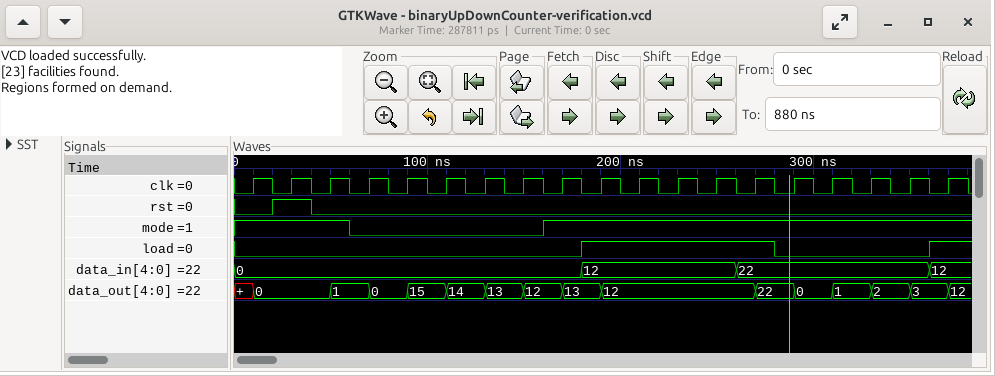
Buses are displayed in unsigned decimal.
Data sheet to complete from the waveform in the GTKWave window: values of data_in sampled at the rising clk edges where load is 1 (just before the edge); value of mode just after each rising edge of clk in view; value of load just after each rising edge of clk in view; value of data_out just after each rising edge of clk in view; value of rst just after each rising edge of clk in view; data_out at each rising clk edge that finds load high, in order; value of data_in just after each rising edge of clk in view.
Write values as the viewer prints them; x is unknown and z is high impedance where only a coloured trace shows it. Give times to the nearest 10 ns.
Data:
12, 12, 12, 12, 22, 12
1 1 1 0 0 0 0 0 1 1 1 1 1 1 1 1 1 1 1
0 0 0 0 0 0 0 0 0 1 1 1 1 1 0 0 0 0 1
0, 0, 1, 0, 15, 14, 13, 12, 13, 12, 12, 12, 12, 22, 0, 1, 2, 3, 12
0 1 0 0 0 0 0 0 0 0 0 0 0 0 0 0 0 0 0
13, 12, 12, 12, 12, 3
0, 0, 0, 0, 0, 0, 0, 0, 0, 12, 12, 12, 12, 22, 22, 22, 22, 22, 12
